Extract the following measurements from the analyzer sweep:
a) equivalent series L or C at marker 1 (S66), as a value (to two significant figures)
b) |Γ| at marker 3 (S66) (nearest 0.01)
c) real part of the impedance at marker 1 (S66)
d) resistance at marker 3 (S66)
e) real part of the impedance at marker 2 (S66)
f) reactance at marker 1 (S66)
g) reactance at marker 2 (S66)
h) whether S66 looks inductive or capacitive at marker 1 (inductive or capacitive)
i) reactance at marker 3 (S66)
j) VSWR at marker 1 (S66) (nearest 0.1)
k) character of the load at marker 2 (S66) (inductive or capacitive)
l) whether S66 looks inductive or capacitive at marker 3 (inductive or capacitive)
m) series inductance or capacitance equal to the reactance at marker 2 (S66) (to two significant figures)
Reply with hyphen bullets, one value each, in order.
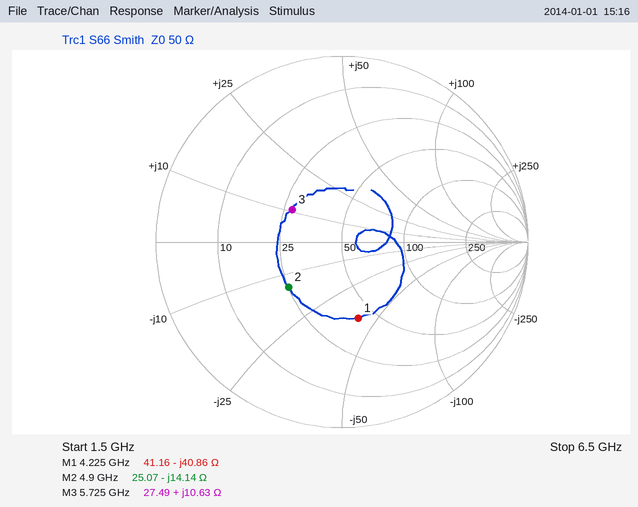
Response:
- 920 fF
- 0.32
- 41.16 Ω
- 27.49 Ω
- 25.07 Ω
- -40.86 Ω
- -14.14 Ω
- capacitive
- +10.63 Ω
- 2.4
- capacitive
- inductive
- 2.3 pF
